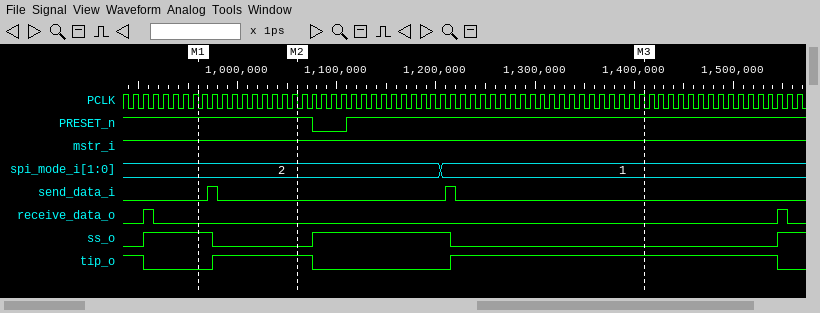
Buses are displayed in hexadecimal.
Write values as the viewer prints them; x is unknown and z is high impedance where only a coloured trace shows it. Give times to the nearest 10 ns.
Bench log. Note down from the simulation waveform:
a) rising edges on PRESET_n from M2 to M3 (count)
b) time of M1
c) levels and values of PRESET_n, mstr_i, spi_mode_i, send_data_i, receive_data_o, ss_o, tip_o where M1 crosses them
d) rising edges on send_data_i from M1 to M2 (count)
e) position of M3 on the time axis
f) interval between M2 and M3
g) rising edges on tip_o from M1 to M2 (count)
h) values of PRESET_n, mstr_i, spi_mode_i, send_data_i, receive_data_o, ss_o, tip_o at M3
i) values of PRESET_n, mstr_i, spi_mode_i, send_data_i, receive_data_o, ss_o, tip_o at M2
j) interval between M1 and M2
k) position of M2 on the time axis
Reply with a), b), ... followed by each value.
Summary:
a) 1
b) 960 ns
c) PRESET_n=1, mstr_i=1, spi_mode_i=2, send_data_i=0, receive_data_o=0, ss_o=1, tip_o=0
d) 1
e) 1410 ns
f) 350 ns
g) 1
h) PRESET_n=1, mstr_i=1, spi_mode_i=1, send_data_i=0, receive_data_o=0, ss_o=0, tip_o=1
i) PRESET_n=1, mstr_i=1, spi_mode_i=2, send_data_i=0, receive_data_o=0, ss_o=0, tip_o=1
j) 100 ns
k) 1060 ns
